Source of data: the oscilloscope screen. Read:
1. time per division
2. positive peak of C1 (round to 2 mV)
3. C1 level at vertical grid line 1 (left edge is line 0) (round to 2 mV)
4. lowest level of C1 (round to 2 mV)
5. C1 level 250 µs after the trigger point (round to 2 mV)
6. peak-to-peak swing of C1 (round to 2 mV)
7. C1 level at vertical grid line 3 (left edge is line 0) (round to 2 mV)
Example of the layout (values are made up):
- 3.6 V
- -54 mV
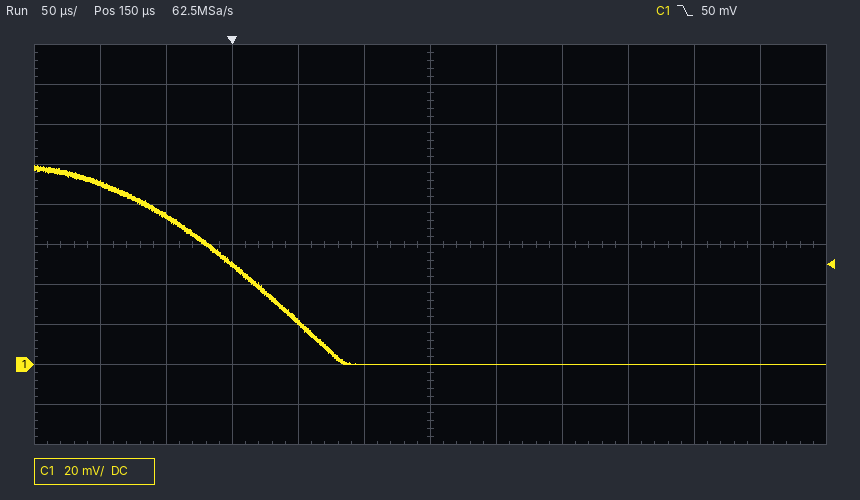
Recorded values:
- 50 µs
- 100 mV
- 90 mV
- 0 mV
- 0 mV
- 100 mV
- 50 mV
